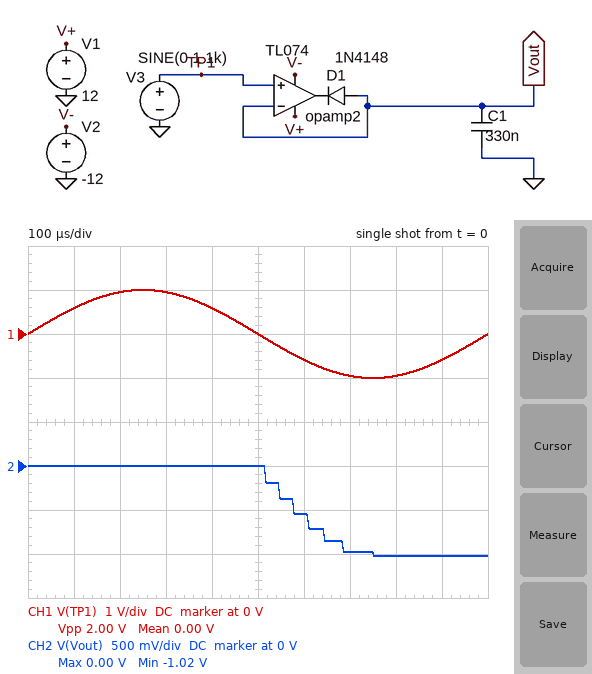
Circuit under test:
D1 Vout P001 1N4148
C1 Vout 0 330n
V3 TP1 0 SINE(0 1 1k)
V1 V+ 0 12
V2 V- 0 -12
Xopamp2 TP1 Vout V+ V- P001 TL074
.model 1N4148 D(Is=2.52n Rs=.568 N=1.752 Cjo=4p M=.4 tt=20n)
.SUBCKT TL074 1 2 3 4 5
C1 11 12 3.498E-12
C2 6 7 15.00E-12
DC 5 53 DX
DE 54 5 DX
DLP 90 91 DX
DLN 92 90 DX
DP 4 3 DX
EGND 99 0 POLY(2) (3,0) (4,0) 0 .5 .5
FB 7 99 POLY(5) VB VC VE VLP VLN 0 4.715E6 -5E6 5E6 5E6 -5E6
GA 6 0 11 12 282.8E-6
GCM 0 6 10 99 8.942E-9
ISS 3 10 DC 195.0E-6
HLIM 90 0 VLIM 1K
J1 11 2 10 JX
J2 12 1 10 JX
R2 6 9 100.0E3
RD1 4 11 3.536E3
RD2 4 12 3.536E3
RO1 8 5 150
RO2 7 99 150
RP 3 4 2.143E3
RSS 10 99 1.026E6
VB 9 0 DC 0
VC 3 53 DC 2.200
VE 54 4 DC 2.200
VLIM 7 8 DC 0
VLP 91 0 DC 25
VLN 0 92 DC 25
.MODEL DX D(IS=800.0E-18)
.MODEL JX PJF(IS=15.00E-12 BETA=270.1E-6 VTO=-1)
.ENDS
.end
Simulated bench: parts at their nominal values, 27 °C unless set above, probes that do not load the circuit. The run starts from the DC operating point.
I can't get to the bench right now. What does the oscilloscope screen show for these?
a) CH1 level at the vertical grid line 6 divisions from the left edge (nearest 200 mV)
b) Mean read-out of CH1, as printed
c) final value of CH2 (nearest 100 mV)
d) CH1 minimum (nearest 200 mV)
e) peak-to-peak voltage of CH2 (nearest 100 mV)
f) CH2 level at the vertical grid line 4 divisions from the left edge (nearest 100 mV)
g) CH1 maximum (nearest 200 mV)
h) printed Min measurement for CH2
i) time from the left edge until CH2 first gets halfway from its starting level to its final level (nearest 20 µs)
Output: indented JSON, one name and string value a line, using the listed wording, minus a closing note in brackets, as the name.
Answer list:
{
  "CH1 level at the vertical grid line 6 divisions from the left edge": "-600 mV",
  "Mean read-out of CH1, as printed": "0.00 V",
  "final value of CH2": "-1.0 V",
  "CH1 minimum": "-1.0 V",
  "peak-to-peak voltage of CH2": "1.0 V",
  "CH2 level at the vertical grid line 4 divisions from the left edge": "0 V",
  "CH1 maximum": "1.0 V",
  "printed Min measurement for CH2": "-1.02 V",
  "time from the left edge until CH2 first gets halfway from its starting level to its final level": "580 µs"
}
